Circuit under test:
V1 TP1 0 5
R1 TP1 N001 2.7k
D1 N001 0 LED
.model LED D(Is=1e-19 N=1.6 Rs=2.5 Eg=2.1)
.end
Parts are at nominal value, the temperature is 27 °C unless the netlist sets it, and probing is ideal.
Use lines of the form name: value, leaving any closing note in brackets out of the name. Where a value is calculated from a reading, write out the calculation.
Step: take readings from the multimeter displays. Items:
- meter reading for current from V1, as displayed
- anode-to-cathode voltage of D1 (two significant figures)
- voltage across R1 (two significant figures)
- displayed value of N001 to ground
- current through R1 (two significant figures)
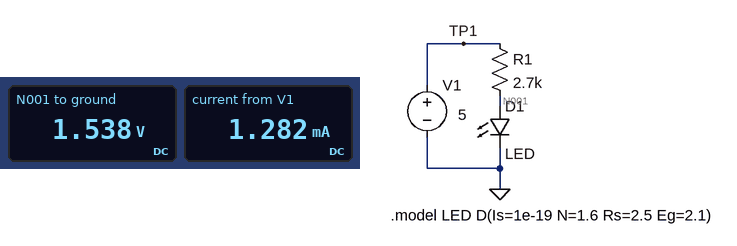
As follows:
meter reading for current from V1, as displayed: 1.282 mA
anode-to-cathode voltage of D1: 1.538 V = 1.5 V
voltage across R1: 5 V - 1.538 V = 3.5 V
displayed value of N001 to ground: 1.538 V
current through R1: (5 V - 1.538 V) / 2.7 kΩ = 1.3 mA
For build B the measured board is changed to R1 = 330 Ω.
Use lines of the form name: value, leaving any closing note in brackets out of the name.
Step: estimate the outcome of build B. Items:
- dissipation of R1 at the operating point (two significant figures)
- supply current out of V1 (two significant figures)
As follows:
dissipation of R1 at the operating point: 34 mW
supply current out of V1: 10 mA
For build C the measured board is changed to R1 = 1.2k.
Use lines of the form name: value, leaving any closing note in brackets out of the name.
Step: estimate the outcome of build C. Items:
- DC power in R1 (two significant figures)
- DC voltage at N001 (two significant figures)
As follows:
DC power in R1: 9.8 mW
DC voltage at N001: 1.6 V
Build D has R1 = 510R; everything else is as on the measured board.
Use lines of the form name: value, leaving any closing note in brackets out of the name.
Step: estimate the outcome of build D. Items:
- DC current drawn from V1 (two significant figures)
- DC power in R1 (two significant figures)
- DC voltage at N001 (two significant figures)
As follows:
DC current drawn from V1: 6.6 mA
DC power in R1: 22 mW
DC voltage at N001: 1.6 V
